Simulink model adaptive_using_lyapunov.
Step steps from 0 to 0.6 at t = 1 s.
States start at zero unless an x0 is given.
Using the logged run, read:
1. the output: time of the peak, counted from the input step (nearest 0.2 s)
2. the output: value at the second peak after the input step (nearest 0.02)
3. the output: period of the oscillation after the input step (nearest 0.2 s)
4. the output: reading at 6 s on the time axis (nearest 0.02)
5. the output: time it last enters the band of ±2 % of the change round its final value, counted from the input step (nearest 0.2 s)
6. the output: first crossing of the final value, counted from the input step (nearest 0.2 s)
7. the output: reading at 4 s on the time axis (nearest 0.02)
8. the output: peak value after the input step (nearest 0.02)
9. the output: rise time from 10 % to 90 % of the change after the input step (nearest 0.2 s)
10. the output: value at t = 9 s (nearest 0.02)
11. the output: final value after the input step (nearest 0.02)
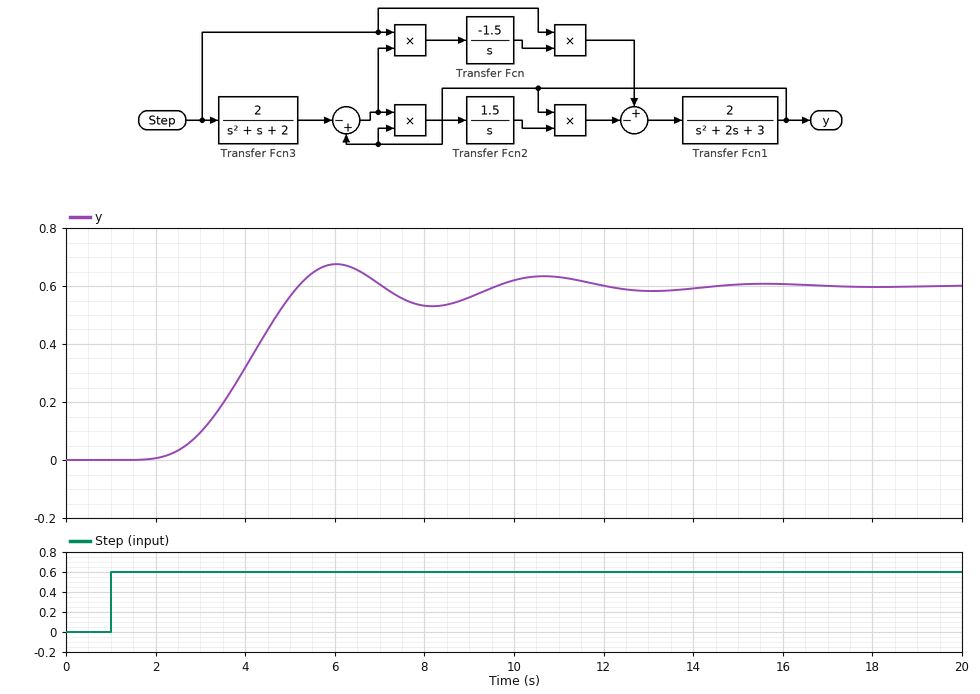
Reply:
5.0 s
0.64
4.6 s
0.68
12.8 s
4.2 s
0.32
0.68
2.2 s
0.56
0.60
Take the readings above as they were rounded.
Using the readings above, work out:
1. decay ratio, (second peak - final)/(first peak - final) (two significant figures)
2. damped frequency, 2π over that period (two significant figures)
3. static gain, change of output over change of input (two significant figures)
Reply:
0.50
1.4 rad/s
1.0
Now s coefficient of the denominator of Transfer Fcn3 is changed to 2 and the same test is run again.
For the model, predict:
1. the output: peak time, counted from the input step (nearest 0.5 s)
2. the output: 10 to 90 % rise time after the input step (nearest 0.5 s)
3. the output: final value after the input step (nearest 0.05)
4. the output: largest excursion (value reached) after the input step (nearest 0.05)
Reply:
6.0 s
3.0 s
0.60
0.65
